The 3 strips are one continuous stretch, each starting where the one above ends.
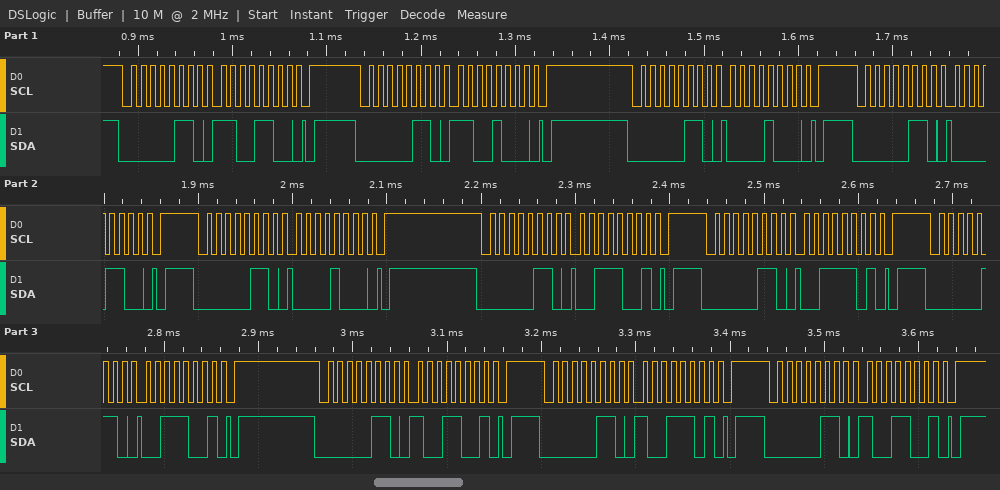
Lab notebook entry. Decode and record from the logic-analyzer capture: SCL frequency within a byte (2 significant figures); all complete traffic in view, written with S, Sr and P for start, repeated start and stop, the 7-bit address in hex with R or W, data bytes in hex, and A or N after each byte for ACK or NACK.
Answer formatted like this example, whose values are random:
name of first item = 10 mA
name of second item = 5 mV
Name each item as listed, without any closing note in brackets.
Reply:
SCL frequency within a byte = 100 kHz
all complete traffic in view, written with S, Sr and P for start, repeated start and stop, the 7-bit address in hex with R or W, data bytes in hex, and A or N after each byte for ACK or NACK = S 03W A CC A P S 03W A C8 A P S 03W A 08 A P S 03W A 0C A P S 03W A 08 A P S 03W A 39 A P S 03W A 3D A P S 03W A 39 A P S 03W A 99 A P S 03W A 9D A P S 03W A 99 A P
